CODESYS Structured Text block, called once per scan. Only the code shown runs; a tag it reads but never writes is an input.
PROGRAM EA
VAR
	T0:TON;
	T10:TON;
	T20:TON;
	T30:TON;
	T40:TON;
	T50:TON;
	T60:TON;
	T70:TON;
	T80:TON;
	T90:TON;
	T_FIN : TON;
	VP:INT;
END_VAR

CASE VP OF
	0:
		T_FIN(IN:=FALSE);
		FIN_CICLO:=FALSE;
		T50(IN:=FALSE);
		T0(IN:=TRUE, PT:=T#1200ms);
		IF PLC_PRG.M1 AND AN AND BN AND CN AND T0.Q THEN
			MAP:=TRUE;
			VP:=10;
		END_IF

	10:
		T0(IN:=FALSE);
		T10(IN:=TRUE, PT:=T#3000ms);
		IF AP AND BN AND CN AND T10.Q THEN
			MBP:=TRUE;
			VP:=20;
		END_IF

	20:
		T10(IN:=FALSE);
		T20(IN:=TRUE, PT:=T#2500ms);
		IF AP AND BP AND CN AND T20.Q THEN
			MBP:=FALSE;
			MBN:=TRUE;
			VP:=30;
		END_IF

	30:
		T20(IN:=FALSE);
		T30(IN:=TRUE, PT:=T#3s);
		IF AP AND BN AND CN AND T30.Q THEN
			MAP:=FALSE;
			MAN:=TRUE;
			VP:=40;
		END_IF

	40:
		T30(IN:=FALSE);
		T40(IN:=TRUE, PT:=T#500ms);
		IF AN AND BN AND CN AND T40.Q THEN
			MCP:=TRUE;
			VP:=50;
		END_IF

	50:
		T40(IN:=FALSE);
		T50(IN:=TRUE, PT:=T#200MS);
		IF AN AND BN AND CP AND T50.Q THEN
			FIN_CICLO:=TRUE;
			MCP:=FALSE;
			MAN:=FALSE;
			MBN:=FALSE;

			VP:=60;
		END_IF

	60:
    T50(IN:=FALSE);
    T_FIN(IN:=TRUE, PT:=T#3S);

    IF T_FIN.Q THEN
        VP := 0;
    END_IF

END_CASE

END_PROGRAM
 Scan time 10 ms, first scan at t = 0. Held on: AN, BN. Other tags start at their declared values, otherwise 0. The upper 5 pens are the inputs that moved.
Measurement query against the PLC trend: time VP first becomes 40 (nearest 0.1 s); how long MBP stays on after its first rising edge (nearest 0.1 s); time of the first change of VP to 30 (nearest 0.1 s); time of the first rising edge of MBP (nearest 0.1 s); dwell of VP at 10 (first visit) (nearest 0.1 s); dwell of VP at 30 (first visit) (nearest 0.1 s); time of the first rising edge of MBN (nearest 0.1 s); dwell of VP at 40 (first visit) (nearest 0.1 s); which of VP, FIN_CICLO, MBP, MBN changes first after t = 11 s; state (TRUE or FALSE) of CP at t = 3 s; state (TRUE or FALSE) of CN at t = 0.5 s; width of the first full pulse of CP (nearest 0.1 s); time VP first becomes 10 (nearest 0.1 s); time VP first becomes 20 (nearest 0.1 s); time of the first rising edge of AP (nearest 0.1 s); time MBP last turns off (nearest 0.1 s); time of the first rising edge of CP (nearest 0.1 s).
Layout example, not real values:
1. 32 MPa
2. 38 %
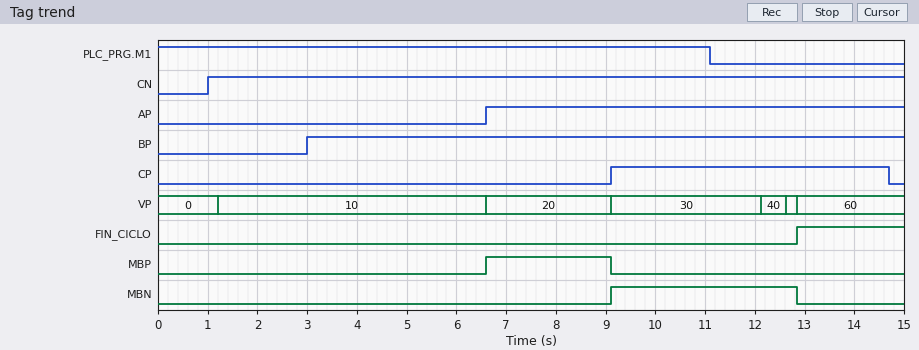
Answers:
1. 12.1 s
2. 2.5 s
3. 9.1 s
4. 6.6 s
5. 5.4 s
6. 3.0 s
7. 9.1 s
8. 0.5 s
9. VP
10. FALSE
11. FALSE
12. 5.6 s
13. 1.2 s
14. 6.6 s
15. 6.6 s
16. 9.1 s
17. 9.1 s
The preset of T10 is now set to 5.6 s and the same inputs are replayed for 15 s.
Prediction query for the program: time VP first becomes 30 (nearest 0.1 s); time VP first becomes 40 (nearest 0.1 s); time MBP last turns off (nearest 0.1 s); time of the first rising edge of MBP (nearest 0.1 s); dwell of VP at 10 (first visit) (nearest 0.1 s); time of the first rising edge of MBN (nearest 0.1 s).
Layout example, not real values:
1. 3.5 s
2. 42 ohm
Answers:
1. 9.3 s
2. 12.3 s
3. 9.3 s
4. 6.8 s
5. 5.6 s
6. 9.3 s
